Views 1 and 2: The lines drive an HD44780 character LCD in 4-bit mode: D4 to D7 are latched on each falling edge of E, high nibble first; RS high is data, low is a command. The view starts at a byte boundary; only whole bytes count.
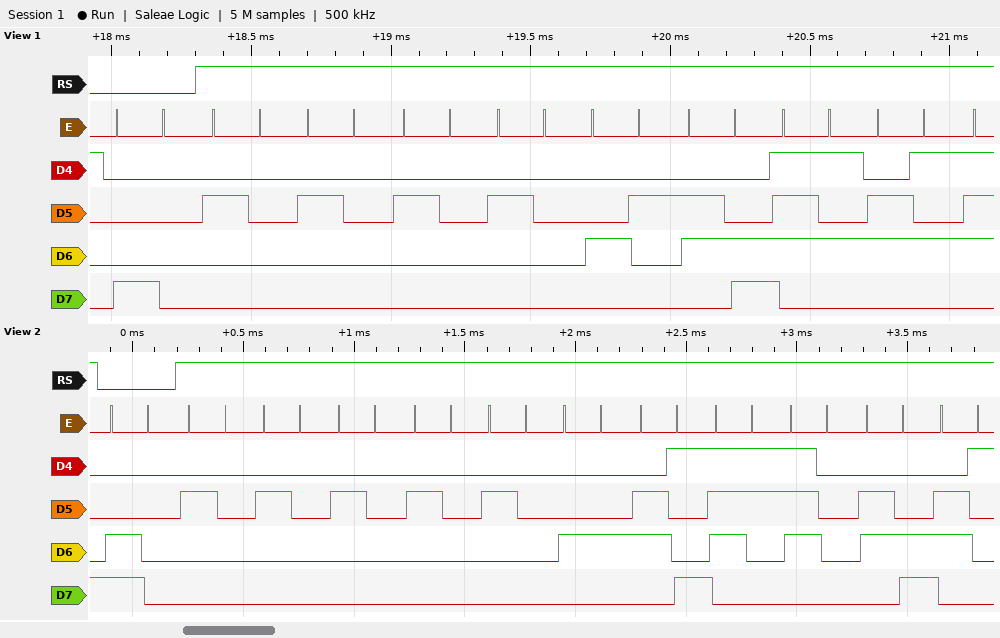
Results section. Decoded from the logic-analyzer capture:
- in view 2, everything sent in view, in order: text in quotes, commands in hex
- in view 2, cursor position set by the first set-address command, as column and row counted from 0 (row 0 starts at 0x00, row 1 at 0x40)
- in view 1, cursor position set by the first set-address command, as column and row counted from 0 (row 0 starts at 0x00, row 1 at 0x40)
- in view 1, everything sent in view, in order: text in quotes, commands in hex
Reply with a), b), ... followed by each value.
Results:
a) 0xC0 "     Displa"
b) column 0, row 1
c) column 0, row 0
d) 0x80 "    Blue"
